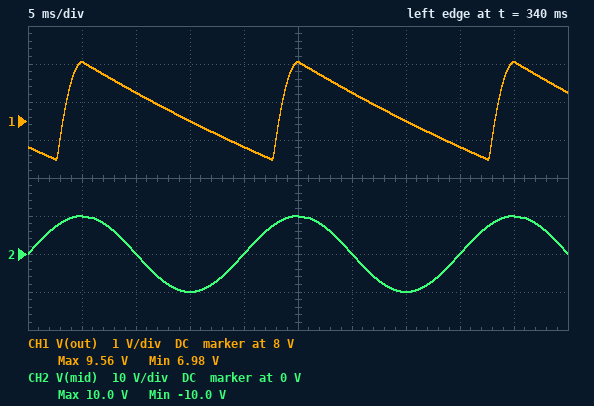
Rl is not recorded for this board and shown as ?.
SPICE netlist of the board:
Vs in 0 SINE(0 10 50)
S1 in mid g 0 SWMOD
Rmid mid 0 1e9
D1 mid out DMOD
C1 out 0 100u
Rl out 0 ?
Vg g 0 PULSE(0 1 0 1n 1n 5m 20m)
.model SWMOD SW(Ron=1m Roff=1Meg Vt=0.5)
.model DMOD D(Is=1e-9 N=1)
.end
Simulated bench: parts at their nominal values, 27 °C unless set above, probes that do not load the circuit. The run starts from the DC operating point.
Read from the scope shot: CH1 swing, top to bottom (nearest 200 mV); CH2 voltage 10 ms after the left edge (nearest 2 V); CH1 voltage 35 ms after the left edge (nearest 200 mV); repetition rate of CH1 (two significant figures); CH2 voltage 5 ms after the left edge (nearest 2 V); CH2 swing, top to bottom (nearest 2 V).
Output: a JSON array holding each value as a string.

["2.6 V", "0 V", "8.0 V", "50 Hz", "10 V", "20 V"]
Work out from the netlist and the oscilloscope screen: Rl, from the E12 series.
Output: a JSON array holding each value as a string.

["560 Ω"]
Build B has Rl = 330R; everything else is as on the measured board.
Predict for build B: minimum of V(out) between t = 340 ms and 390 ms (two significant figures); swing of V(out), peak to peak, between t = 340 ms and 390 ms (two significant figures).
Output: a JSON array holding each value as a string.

["5.7 V", "3.9 V"]
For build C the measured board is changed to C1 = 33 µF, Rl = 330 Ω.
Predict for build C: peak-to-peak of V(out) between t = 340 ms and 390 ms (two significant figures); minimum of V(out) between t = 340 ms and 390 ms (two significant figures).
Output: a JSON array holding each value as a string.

["7.3 V", "2.2 V"]
